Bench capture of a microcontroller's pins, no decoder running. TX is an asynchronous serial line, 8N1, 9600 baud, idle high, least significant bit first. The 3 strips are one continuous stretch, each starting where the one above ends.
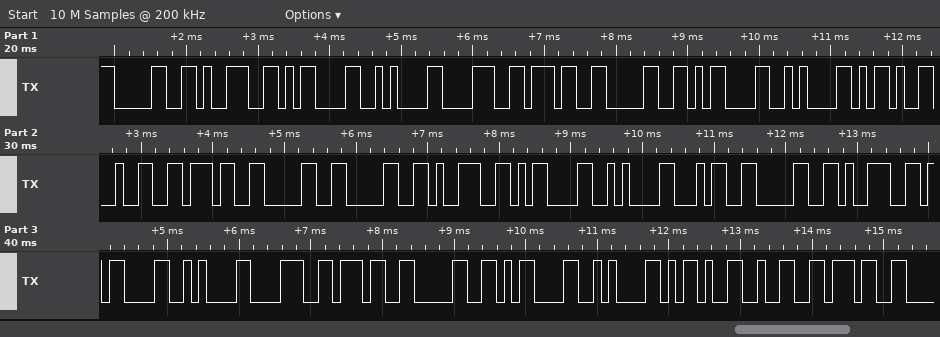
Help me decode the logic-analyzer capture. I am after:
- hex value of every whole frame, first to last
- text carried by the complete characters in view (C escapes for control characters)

0x30 0x39 0x0D 0x0A 0x38 0x37 0x30 0x0D 0x0A 0x2D 0x32 0x37 0x30 0x30 0x39 0x0D 0x0A 0x34 0x30 0x39 0x0D 0x0A 0x38 0x37 0x30 0x0D 0x0A 0x2D 0x32 0x37
"09\r\n870\r\n-27009\r\n409\r\n870\r\n-27"
